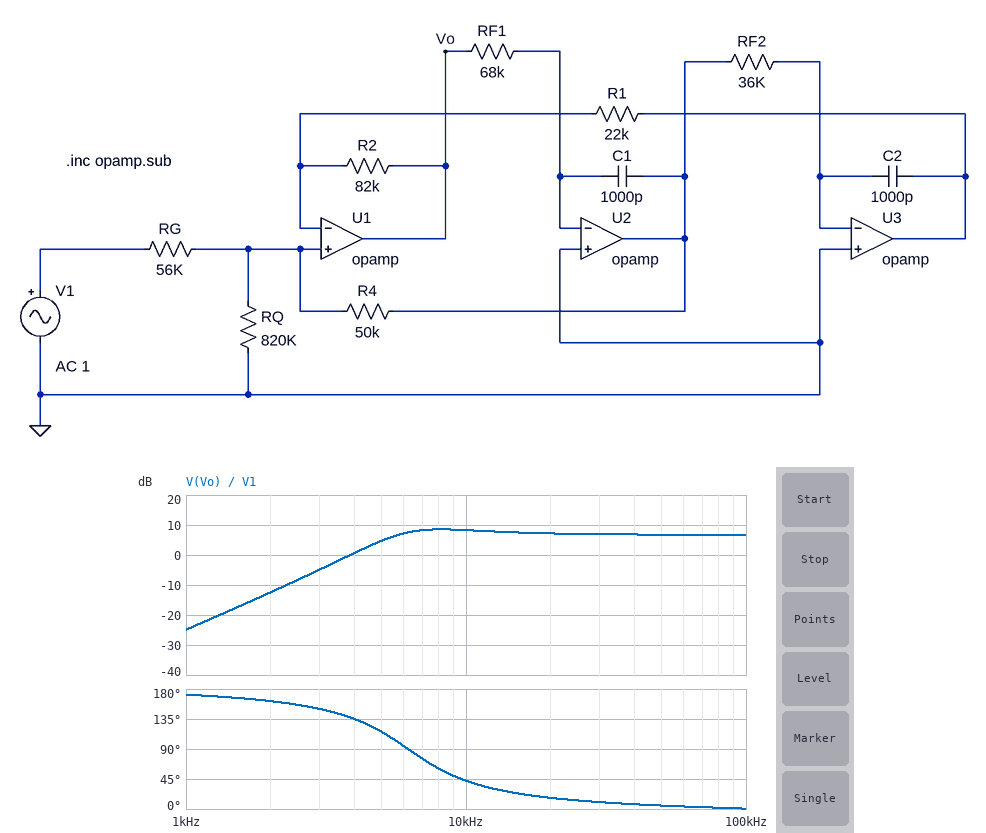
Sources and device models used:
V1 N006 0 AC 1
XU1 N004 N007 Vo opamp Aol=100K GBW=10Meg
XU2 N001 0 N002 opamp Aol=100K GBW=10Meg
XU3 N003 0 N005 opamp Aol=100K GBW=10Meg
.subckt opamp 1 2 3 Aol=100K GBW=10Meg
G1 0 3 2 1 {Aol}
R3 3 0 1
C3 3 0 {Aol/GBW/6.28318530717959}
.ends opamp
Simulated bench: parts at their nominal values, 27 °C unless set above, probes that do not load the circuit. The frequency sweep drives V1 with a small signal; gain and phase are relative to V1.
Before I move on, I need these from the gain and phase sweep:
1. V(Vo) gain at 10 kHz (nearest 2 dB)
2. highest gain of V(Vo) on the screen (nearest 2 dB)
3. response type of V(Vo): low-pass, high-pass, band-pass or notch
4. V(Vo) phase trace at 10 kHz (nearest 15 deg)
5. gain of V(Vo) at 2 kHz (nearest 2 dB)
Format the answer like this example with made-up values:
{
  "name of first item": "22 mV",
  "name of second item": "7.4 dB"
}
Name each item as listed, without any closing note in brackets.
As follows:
{
  "V(Vo) gain at 10 kHz": "8 dB",
  "highest gain of V(Vo) on the screen": "8 dB",
  "response type of V(Vo): low-pass, high-pass, band-pass or notch": "high-pass",
  "V(Vo) phase trace at 10 kHz": "45 deg",
  "gain of V(Vo) at 2 kHz": "-12 dB"
}
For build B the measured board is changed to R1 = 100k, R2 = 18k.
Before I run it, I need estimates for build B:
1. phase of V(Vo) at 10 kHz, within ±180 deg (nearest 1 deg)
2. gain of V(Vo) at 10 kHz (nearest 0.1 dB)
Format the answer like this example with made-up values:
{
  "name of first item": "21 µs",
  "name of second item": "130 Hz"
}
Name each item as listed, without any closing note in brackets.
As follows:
{
  "phase of V(Vo) at 10 kHz, within ±180 deg": "8 deg",
  "gain of V(Vo) at 10 kHz": "-5.3 dB"
}
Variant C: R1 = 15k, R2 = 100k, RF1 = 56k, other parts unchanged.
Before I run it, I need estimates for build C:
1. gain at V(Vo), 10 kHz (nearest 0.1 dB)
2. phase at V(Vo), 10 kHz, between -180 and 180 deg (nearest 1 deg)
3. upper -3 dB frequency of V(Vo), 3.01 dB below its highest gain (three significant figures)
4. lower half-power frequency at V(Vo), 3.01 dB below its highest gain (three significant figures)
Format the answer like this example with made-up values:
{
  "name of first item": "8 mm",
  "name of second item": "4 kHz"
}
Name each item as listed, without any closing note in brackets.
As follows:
{
  "gain at V(Vo), 10 kHz": "9.9 dB",
  "phase at V(Vo), 10 kHz, between -180 and 180 deg": "82 deg",
  "upper -3 dB frequency of V(Vo), 3.01 dB below its highest gain": "1.20 MHz",
  "lower half-power frequency at V(Vo), 3.01 dB below its highest gain": "8.30 kHz"
}
